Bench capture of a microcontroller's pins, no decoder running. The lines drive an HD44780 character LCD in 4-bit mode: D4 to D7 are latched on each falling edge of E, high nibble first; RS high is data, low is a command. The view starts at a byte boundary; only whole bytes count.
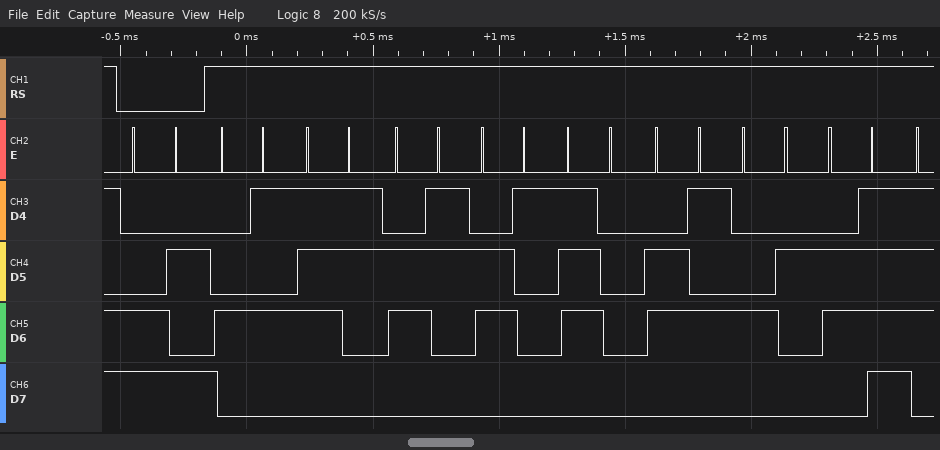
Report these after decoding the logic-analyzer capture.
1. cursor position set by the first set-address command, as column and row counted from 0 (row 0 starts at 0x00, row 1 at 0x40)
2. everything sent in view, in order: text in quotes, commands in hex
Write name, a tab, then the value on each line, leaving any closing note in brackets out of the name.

cursor position set by the first set-address command, as column and row counted from 0	column 10, row 1
everything sent in view, in order: text in quotes, commands in hex	0xCA "EscapeBo"
